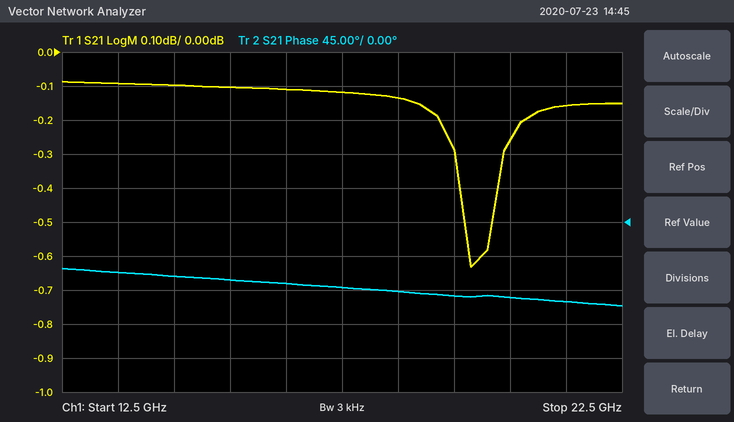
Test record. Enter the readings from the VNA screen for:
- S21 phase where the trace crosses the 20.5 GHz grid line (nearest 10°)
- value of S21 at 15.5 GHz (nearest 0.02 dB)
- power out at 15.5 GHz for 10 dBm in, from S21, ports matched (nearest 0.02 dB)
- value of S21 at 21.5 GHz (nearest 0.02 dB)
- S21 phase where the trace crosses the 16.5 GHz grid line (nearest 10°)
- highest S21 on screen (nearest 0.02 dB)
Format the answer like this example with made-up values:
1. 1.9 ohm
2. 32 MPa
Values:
1. -100°
2. -0.10 dB
3. 9.90 dBm
4. -0.16 dB
5. -80°
6. -0.08 dB
